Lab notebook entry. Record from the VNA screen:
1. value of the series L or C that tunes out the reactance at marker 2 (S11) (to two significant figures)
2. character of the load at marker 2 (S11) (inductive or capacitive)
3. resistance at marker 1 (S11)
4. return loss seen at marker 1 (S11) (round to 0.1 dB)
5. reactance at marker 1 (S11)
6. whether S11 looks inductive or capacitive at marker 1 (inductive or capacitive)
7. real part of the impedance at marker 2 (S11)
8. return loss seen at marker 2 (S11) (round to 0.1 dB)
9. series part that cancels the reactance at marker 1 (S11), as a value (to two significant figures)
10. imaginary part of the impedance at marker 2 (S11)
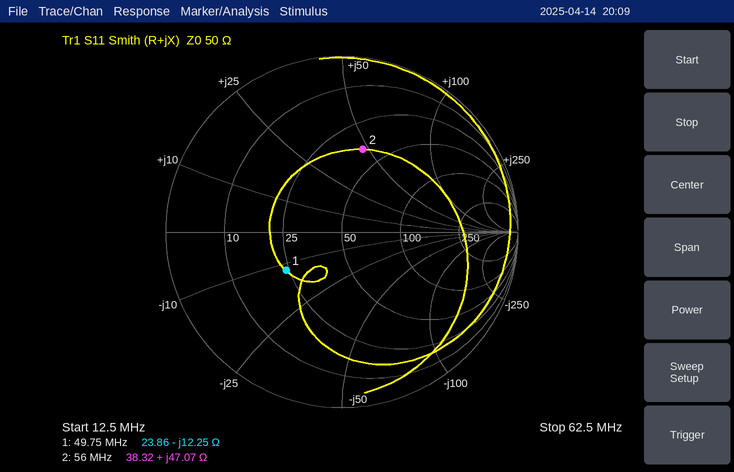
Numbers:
60 pF
inductive
23.86 Ω
8.3 dB
-12.25 Ω
capacitive
38.32 Ω
6.3 dB
39 nH
+47.07 Ω
